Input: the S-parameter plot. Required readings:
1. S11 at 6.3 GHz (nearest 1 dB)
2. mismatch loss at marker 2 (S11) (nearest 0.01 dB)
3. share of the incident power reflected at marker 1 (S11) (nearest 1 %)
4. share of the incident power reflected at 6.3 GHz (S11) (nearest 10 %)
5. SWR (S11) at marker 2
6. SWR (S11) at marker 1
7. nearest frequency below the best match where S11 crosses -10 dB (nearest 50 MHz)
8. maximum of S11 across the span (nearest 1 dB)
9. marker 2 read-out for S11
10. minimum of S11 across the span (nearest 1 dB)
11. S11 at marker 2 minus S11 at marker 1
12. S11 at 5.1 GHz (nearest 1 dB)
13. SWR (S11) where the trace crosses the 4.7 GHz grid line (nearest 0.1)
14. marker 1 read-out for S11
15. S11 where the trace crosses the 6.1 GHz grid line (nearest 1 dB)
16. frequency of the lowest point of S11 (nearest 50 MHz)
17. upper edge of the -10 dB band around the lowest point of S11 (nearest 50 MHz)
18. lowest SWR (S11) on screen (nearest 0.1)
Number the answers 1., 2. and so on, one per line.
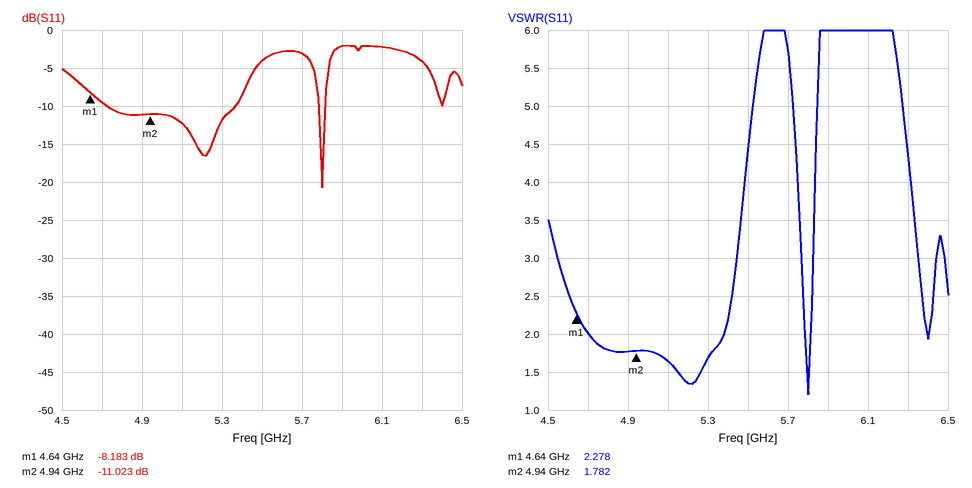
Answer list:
1. -4 dB
2. 0.36 dB
3. 15 %
4. 40 %
5. 1.782
6. 2.278
7. 5.80 GHz
8. -2 dB
9. -11.023 dB
10. -21 dB
11. -2.840 dB
12. -12 dB
13. 2.0
14. -8.183 dB
15. -2 dB
16. 5.80 GHz
17. 5.80 GHz
18. 1.2
